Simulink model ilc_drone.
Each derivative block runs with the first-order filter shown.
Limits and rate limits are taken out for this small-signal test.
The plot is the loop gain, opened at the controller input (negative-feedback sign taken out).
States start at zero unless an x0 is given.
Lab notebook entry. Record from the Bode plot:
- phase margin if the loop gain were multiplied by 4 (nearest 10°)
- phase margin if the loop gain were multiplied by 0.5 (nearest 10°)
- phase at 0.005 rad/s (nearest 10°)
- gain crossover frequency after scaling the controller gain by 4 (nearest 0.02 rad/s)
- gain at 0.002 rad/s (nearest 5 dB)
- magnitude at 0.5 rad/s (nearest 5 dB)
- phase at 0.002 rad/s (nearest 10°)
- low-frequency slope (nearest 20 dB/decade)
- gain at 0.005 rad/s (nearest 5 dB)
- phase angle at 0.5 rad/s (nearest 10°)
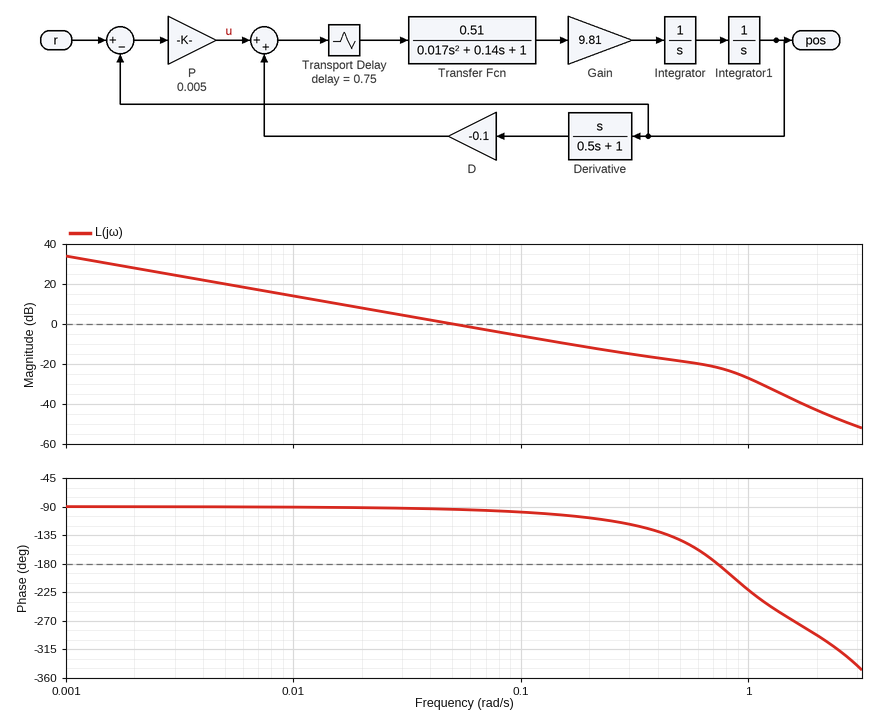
70°
90°
-90°
0.20 rad/s
30 dB
-20 dB
-90°
-20 dB/decade
20 dB
-140°
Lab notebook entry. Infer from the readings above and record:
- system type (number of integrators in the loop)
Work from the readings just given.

1
